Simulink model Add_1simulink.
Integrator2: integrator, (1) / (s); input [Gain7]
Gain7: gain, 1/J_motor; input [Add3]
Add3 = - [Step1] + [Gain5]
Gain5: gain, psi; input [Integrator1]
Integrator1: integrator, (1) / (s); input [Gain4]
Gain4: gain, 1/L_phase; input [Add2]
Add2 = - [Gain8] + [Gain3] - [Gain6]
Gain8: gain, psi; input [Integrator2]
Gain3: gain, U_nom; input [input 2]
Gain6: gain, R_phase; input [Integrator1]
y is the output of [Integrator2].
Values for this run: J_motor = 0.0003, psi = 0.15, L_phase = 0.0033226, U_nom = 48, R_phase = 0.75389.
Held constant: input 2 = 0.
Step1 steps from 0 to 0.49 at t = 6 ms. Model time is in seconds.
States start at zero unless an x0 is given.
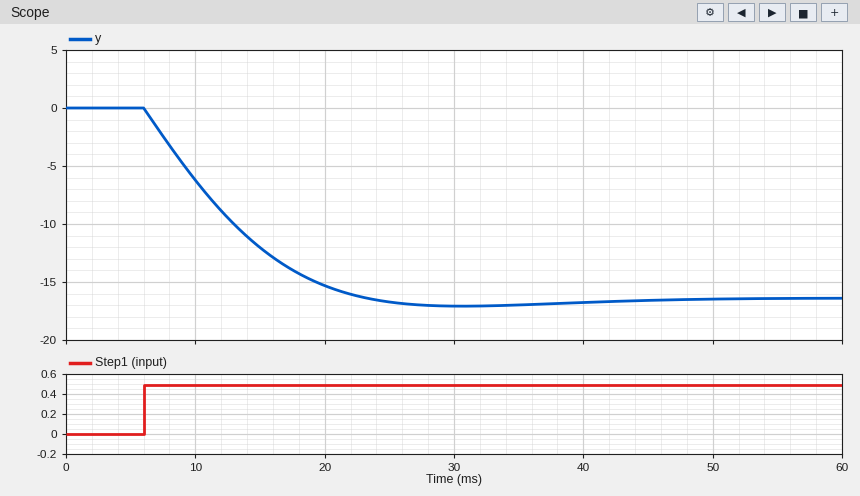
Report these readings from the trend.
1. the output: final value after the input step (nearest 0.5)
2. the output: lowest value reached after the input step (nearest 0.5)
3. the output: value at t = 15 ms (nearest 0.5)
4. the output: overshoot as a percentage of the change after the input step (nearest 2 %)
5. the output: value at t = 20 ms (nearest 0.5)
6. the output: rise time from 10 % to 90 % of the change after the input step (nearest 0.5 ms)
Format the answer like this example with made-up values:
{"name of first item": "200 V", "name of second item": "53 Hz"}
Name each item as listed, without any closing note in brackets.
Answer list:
{"the output: final value after the input step": "-16.5", "the output: lowest value reached after the input step": "-17.0", "the output: value at t = 15 ms": "-12.0", "the output: overshoot as a percentage of the change after the input step": "4 %", "the output: value at t = 20 ms": "-15.5", "the output: rise time from 10 % to 90 % of the change after the input step": "12.0 ms"}
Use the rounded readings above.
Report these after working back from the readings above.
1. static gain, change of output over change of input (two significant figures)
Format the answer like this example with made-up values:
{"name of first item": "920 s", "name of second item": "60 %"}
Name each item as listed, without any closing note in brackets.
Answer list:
{"static gain, change of output over change of input": "-34"}
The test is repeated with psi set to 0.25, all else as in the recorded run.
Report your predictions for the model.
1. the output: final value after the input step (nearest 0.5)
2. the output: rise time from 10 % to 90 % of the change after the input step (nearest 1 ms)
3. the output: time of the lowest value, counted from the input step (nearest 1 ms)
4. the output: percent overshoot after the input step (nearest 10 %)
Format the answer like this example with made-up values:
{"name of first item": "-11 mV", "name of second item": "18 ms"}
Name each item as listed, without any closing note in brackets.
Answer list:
{"the output: final value after the input step": "-6.0", "the output: rise time from 10 % to 90 % of the change after the input step": "3 ms", "the output: time of the lowest value, counted from the input step": "9 ms", "the output: percent overshoot after the input step": "40 %"}
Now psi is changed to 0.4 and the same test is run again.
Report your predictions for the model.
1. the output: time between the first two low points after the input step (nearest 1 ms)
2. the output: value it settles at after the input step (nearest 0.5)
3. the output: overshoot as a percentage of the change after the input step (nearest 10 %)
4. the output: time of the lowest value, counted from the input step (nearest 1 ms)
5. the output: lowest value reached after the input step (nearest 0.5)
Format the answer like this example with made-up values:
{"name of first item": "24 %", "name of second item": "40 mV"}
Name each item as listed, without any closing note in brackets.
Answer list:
{"the output: time between the first two low points after the input step": "16 ms", "the output: value it settles at after the input step": "-2.5", "the output: overshoot as a percentage of the change after the input step": "100 %", "the output: time of the lowest value, counted from the input step": "5 ms", "the output: lowest value reached after the input step": "-4.5"}
